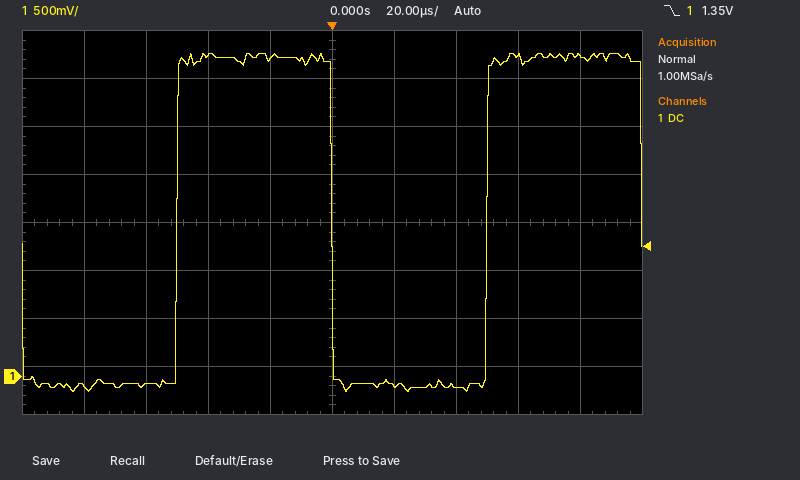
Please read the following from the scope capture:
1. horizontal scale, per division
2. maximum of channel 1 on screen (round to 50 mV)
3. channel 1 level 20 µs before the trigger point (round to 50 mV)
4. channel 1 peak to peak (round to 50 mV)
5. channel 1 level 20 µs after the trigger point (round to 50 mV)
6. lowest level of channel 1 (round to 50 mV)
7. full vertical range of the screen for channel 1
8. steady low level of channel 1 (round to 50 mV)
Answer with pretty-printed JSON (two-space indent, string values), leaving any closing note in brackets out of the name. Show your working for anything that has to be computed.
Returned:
{
  "horizontal scale, per division": "20 µs",
  "maximum of channel 1 on screen": "3.35 V",
  "channel 1 level 20 µs before the trigger point": "3.30 V",
  "channel 1 peak to peak": "3.35 V − (-150 mV) = 3.50 V",
  "channel 1 level 20 µs after the trigger point": "-100 mV",
  "lowest level of channel 1": "-150 mV",
  "full vertical range of the screen for channel 1": "4 V",
  "steady low level of channel 1": "-100 mV"
}
